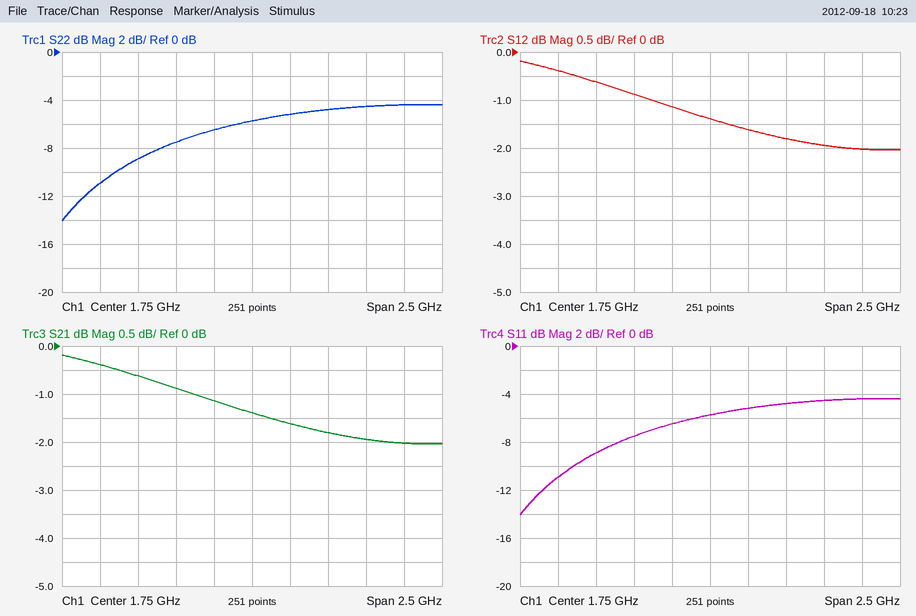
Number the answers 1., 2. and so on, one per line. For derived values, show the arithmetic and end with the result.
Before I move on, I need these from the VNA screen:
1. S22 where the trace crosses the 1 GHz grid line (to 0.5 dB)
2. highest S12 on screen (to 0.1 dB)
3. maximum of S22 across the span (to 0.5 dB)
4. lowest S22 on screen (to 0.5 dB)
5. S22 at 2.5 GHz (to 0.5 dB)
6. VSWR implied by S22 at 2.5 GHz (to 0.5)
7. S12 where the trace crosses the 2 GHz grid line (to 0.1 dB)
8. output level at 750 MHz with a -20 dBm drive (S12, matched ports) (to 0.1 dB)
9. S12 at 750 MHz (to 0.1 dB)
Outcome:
1. -9.0 dB
2. -0.2 dB
3. -4.5 dB
4. -14.0 dB
5. -4.5 dB
6. |Γ| = 10^(-4.5/20) = 0.5957; VSWR = (1 + 0.5957)/(1 − 0.5957) ≈ 4.0
7. -1.6 dB
8. -20 dBm + (-0.4 dB) = -20.4 dBm
9. -0.4 dB
